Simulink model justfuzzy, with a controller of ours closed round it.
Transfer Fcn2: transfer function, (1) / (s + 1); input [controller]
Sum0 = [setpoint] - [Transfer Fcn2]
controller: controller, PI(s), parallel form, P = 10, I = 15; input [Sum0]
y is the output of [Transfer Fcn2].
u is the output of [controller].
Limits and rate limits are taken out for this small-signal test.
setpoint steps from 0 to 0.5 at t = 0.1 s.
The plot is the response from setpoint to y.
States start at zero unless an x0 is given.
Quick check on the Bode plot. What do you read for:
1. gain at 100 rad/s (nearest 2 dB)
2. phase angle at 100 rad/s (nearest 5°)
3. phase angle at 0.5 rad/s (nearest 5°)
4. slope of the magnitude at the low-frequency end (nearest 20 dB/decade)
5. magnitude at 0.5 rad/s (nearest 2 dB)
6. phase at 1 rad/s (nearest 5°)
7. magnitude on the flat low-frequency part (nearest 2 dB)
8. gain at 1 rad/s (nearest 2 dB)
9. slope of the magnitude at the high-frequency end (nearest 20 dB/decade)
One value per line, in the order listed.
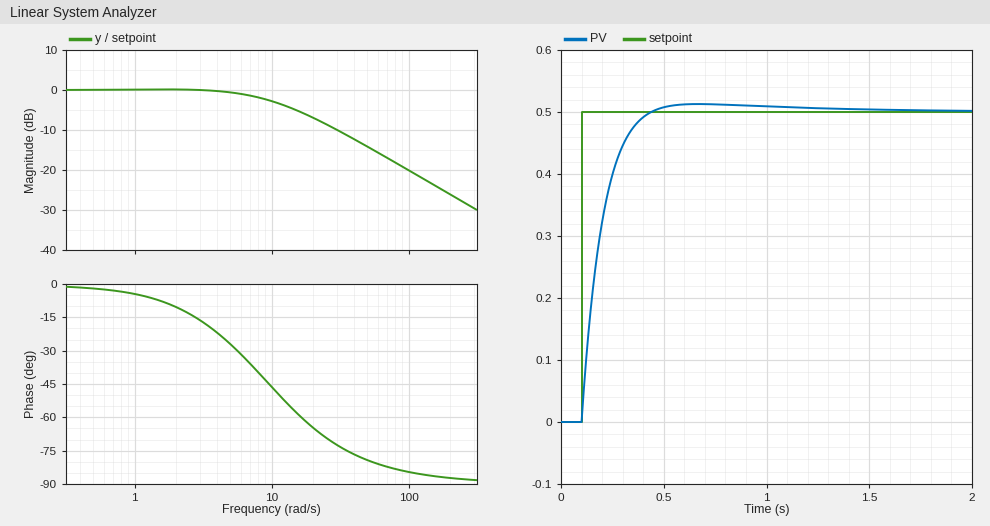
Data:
-20 dB
-85°
0°
0 dB/decade
0 dB
-5°
0 dB
0 dB
-20 dB/decade
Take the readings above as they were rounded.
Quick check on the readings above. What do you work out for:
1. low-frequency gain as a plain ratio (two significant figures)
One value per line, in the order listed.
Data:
1.0
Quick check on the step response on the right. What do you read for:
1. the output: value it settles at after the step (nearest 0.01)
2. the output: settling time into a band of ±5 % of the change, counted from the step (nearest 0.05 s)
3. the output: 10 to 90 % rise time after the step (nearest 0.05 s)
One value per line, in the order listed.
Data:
0.50
0.25 s
0.20 s
